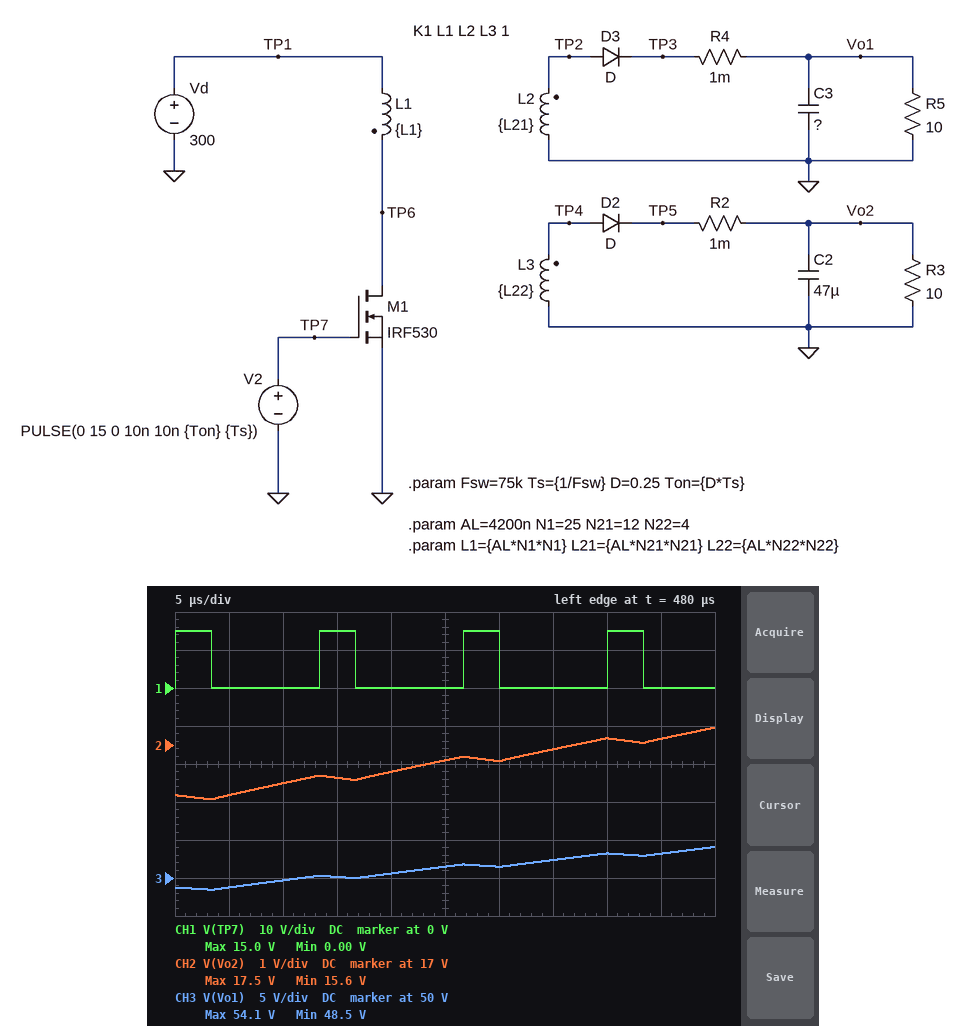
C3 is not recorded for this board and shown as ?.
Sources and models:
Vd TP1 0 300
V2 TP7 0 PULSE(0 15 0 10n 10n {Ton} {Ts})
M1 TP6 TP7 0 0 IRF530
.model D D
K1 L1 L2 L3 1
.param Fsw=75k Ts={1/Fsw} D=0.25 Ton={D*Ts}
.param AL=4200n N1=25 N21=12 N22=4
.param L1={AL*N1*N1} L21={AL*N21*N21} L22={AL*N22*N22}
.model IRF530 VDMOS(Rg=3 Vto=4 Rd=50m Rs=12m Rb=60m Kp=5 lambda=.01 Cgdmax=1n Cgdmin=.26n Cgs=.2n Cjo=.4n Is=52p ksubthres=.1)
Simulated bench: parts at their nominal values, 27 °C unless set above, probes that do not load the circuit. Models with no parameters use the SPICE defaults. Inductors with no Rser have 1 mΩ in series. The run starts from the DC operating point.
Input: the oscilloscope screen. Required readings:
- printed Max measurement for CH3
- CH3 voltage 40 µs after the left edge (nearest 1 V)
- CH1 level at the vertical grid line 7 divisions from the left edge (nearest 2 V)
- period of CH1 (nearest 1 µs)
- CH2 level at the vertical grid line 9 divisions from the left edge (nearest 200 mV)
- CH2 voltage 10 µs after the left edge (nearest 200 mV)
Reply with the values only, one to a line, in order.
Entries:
54.1 V
53 V
0 V
13 µs
17.2 V
16.0 V
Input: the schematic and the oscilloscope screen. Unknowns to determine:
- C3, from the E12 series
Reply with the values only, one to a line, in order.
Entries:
56 µF
